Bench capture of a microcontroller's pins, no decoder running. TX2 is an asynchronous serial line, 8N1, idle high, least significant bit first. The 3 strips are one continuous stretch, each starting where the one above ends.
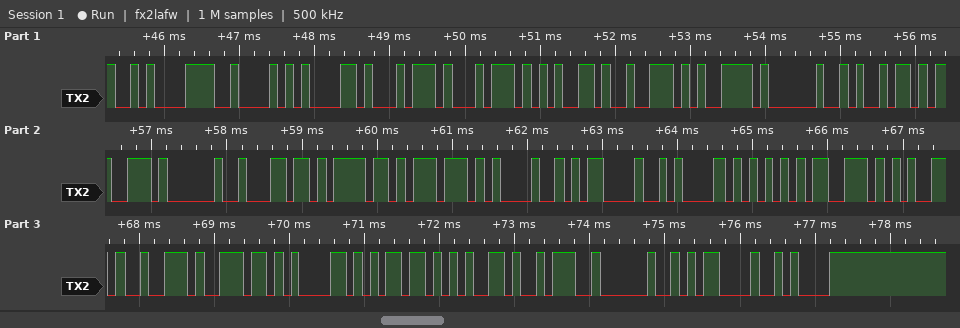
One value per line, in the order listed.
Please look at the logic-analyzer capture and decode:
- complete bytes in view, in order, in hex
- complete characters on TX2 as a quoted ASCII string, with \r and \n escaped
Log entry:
0x0A 0x42 0x61 0x74 0x74 0x65 0x72 0x79 0x20 0x69 0x73 0x20 0x6C 0x6F 0x77 0x21 0x0D 0x0A 0x55 0x73 0x65 0x72 0x6E 0x61 0x6D 0x65 0x3A 0x20 0x0D 0x0A
"\nBattery is low!\r\nUsername: \r\n"
